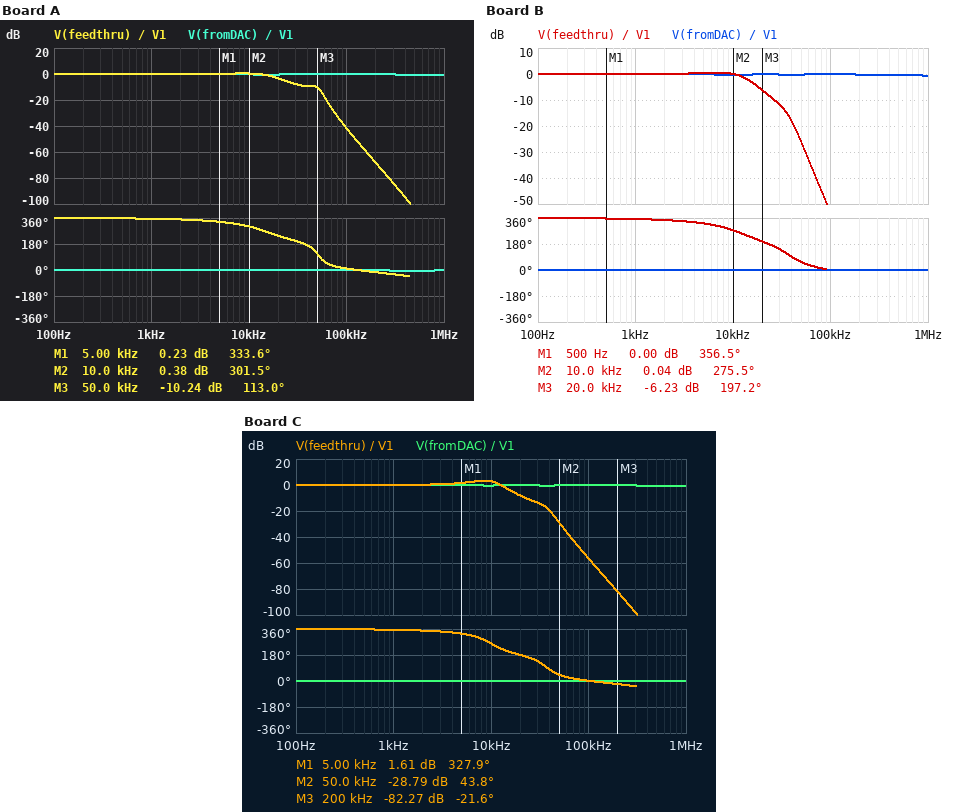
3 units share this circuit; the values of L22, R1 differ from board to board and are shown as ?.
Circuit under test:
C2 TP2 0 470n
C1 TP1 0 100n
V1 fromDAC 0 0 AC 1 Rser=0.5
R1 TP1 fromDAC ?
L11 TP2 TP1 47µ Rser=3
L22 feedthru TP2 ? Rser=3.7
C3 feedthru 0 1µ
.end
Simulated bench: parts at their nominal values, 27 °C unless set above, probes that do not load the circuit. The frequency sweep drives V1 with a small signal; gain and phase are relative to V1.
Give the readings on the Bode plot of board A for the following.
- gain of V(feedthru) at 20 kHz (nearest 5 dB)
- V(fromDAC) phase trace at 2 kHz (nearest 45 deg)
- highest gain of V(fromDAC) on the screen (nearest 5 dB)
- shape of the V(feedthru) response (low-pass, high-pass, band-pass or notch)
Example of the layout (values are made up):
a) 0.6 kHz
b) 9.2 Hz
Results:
a) -5 dB
b) 0 deg
c) 0 dB
d) low-pass
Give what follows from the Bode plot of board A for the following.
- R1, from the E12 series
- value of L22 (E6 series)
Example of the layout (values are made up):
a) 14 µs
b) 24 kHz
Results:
a) 3.3 Ω
b) 47 µH
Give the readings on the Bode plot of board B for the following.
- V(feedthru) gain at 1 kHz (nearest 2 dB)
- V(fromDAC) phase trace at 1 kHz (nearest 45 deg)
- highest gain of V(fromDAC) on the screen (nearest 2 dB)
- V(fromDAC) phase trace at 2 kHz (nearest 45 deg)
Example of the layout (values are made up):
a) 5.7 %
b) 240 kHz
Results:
a) 0 dB
b) 0 deg
c) 0 dB
d) 0 deg
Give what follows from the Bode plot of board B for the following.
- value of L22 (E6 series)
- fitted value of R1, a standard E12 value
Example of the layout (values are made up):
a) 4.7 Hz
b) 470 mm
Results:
a) 150 µH
b) 6.8 Ω
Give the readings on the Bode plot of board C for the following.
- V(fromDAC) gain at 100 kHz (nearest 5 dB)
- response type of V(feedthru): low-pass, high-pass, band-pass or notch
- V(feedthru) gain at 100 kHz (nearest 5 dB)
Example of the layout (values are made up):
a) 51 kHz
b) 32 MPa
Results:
a) 0 dB
b) low-pass
c) -55 dB
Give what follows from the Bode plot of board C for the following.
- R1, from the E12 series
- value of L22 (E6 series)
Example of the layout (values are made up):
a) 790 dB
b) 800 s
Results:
a) 3.9 Ω
b) 220 µH
